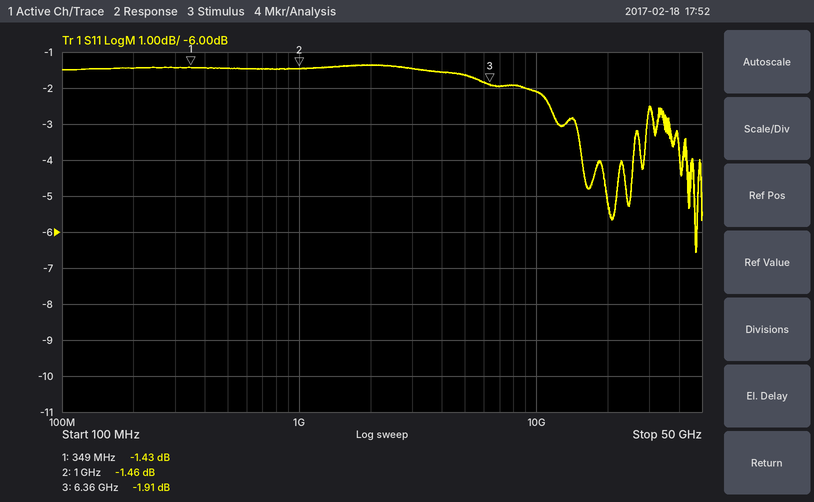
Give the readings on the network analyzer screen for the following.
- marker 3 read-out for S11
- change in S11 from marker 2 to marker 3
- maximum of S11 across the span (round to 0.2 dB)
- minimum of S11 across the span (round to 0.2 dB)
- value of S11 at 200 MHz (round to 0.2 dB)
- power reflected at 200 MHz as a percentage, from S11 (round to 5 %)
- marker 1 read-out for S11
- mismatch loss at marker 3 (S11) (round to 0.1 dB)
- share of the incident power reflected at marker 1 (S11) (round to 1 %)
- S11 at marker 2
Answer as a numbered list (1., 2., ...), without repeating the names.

1. -1.91 dB
2. -0.45 dB
3. -1.4 dB
4. -6.6 dB
5. -1.4 dB
6. 70 %
7. -1.43 dB
8. 4.5 dB
9. 72 %
10. -1.46 dB
